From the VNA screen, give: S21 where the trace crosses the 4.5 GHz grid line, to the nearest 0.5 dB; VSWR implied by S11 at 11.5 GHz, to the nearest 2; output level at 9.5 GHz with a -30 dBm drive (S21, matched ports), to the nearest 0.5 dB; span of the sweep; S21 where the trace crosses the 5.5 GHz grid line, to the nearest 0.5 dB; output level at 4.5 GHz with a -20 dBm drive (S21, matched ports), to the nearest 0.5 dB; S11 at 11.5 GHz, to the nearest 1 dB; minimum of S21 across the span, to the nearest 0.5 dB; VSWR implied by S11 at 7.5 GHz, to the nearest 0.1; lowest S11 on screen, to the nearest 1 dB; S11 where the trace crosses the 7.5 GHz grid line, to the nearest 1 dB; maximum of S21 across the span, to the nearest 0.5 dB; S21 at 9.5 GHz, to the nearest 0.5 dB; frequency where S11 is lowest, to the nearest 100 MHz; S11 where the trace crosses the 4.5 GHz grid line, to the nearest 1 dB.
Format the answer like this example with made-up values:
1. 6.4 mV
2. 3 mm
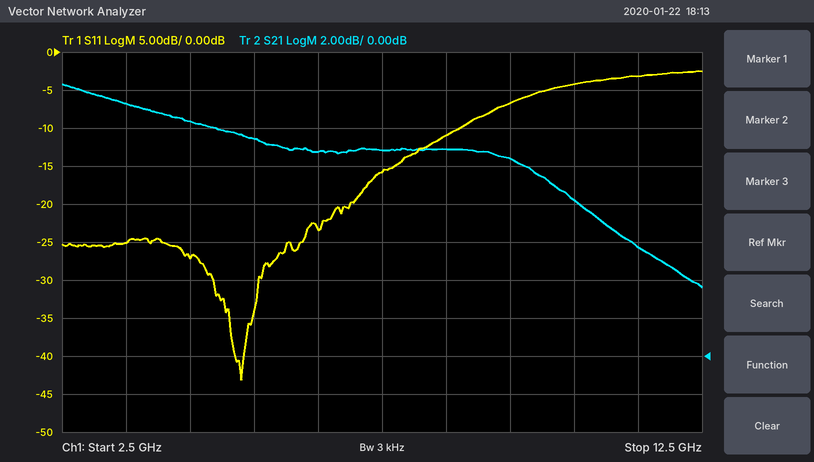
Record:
1. 12.5 dB
2. 6
3. -19.5 dBm
4. 10 GHz
5. 11.5 dB
6. -7.5 dBm
7. -3 dB
8. 3.5 dB
9. 1.4
10. -43 dB
11. -16 dB
12. 14.5 dB
13. 10.5 dB
14. 5.3 GHz
15. -27 dB
